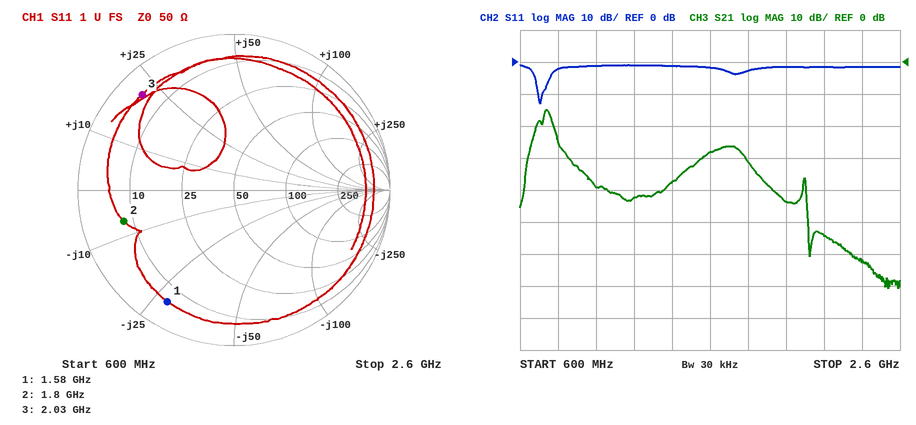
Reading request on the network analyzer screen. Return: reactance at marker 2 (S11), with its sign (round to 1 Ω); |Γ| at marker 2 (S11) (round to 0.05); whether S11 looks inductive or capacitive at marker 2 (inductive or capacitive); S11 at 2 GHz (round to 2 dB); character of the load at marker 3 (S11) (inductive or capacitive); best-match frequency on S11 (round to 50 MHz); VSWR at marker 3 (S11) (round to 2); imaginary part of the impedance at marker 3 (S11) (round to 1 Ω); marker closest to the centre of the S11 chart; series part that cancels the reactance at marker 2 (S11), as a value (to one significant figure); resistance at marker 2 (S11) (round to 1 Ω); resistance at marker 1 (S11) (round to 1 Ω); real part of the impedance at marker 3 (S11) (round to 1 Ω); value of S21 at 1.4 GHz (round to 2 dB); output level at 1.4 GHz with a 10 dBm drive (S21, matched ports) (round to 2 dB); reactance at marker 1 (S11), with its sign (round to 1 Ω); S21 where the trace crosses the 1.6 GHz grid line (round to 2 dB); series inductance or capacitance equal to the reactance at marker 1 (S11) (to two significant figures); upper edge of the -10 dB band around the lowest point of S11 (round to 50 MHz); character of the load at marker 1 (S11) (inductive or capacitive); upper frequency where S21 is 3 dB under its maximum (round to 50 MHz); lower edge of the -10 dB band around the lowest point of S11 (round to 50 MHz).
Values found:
-7 Ω
0.75
capacitive
-2 dB
inductive
700 MHz
12
+21 Ω
marker 2
600 pH
8 Ω
6 Ω
5 Ω
-38 dB
-28 dBm
-28 Ω
-28 dB
3.6 pF
700 MHz
capacitive
750 MHz
700 MHz
